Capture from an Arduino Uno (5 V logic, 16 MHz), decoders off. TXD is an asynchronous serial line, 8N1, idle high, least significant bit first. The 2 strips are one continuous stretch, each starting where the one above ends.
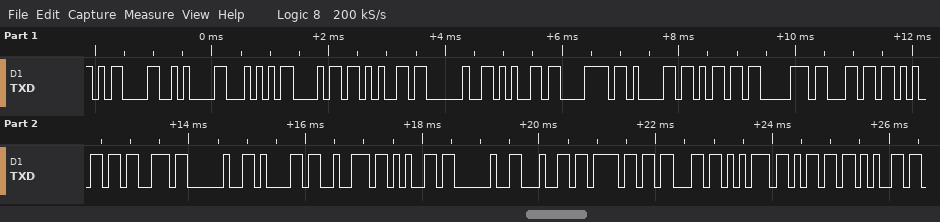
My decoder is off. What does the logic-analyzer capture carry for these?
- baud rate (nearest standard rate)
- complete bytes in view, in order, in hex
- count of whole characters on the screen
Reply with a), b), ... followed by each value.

a) 9600 baud
b) 0D 0A 54 68 65 20 65 78 61 6D 70 6C 65 73 20 61 72 65 20 64 6F 63 75 6D 65
c) 25
